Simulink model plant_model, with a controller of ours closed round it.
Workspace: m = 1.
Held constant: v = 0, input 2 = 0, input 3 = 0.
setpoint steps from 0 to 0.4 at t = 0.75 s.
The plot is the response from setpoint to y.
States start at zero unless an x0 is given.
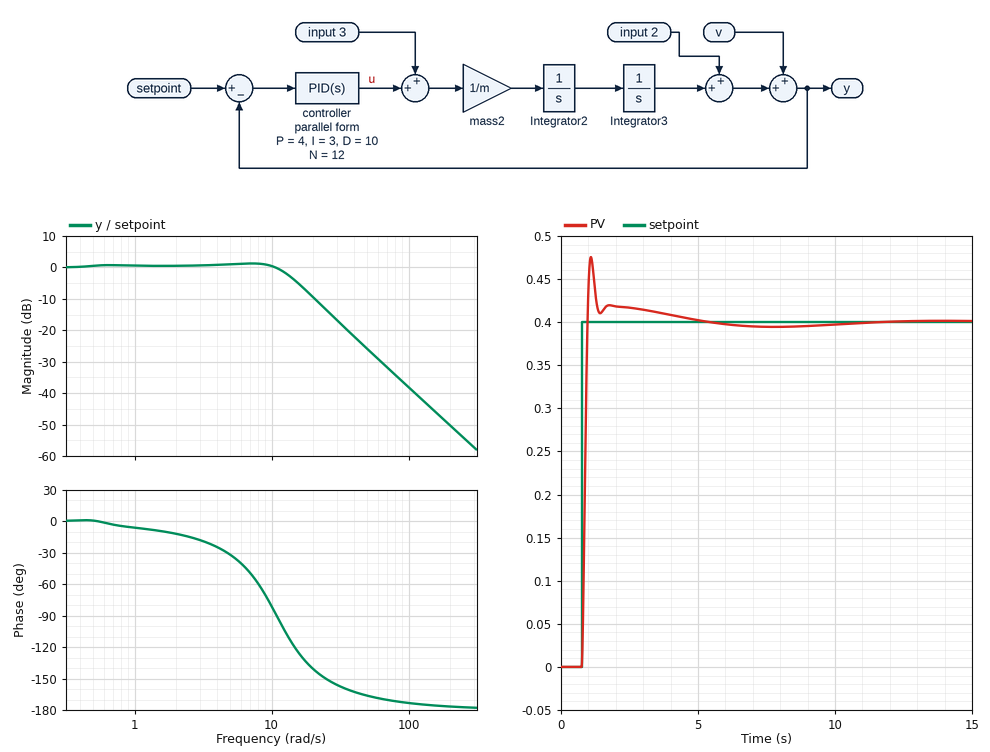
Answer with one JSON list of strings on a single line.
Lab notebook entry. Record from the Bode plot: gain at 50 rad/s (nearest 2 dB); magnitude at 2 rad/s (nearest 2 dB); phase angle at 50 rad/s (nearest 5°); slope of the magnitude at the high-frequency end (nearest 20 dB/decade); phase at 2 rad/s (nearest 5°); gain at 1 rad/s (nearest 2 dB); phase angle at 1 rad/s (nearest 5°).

["-26 dB", "0 dB", "-165°", "-40 dB/decade", "-10°", "0 dB", "-5°"]
